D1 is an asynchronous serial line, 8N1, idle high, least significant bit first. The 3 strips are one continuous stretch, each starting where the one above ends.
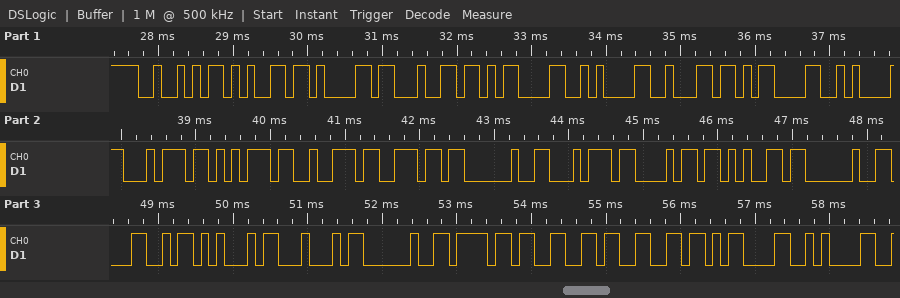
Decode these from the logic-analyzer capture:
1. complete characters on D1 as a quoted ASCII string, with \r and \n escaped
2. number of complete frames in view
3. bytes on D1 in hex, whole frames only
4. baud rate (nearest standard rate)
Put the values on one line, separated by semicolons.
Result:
"Read\r\nb\r\nturn the LED off\r\n"; 27; 52 65 61 64 0D 0A 62 0D 0A 74 75 72 6E 20 74 68 65 20 4C 45 44 20 6F 66 66 0D 0A; 9600 baud
